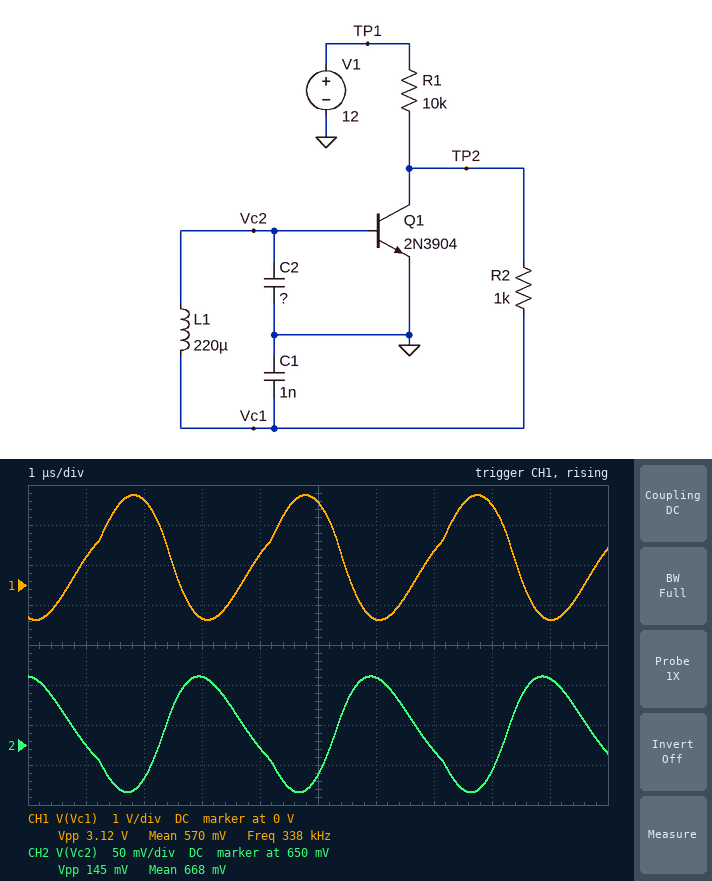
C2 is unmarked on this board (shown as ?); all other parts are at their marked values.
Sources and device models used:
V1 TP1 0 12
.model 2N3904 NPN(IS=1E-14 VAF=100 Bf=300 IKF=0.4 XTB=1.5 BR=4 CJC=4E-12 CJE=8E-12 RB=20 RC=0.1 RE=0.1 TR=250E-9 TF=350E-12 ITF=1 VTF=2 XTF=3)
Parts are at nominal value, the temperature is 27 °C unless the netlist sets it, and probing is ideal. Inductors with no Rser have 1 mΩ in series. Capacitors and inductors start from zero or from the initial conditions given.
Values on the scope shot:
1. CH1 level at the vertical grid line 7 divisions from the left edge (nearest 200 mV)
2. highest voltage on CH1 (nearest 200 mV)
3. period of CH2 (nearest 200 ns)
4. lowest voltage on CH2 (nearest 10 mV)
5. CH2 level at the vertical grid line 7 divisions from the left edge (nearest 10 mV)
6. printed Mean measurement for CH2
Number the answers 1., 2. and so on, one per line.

1. 800 mV
2. 2.2 V
3. 3.0 µs
4. 590 mV
5. 640 mV
6. 668 mV
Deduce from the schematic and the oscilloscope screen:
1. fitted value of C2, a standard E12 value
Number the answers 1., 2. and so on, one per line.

1. 18 nF
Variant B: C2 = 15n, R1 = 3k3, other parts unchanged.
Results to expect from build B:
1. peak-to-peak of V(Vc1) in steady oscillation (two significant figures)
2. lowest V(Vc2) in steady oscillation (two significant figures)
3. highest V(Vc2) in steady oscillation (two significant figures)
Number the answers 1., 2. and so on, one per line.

1. 5.2 V
2. 570 mV
3. 820 mV
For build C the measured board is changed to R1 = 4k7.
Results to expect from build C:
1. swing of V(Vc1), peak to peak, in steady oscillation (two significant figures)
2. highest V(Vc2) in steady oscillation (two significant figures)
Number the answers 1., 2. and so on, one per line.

1. 4.3 V
2. 780 mV
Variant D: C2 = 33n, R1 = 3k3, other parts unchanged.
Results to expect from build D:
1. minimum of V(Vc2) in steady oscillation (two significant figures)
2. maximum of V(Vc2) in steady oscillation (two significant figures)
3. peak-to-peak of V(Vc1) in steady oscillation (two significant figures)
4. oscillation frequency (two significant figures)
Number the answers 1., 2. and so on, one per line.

1. 650 mV
2. 750 mV
3. 3.9 V
4. 330 kHz
